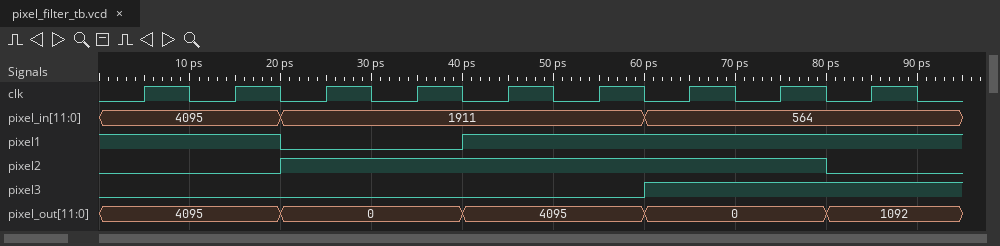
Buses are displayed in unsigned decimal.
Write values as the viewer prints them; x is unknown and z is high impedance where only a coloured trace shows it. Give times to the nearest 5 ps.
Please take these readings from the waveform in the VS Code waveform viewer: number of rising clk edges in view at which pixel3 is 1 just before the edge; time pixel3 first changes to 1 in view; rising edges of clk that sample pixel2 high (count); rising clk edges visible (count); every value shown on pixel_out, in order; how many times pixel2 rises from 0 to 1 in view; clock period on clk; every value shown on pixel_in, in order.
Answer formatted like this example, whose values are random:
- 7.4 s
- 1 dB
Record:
- 3
- 60 ps
- 6
- 9
- 4095, 0, 4095, 0, 1092
- 1
- 10 ps
- 4095, 1911, 564
